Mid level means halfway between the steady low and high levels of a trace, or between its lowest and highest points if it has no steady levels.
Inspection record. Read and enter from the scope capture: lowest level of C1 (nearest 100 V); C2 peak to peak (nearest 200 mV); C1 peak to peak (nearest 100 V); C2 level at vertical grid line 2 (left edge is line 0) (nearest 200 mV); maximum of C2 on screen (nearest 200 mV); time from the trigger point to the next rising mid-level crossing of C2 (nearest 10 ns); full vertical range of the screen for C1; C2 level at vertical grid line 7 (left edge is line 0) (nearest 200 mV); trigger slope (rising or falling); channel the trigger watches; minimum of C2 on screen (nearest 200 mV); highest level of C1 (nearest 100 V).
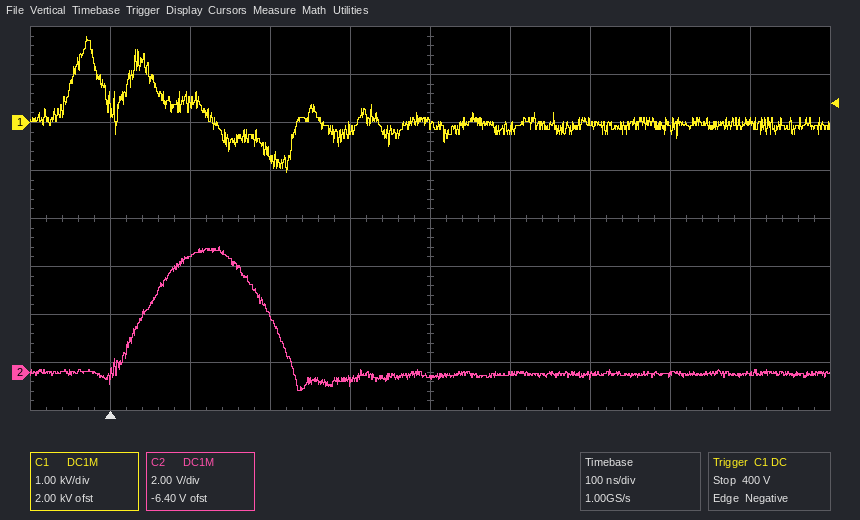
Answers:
-1.0 kV
6.0 V
2.8 kV
4.8 V
5.2 V
40 ns
8 kV
-200 mV
falling
C1
-800 mV
1.8 kV
